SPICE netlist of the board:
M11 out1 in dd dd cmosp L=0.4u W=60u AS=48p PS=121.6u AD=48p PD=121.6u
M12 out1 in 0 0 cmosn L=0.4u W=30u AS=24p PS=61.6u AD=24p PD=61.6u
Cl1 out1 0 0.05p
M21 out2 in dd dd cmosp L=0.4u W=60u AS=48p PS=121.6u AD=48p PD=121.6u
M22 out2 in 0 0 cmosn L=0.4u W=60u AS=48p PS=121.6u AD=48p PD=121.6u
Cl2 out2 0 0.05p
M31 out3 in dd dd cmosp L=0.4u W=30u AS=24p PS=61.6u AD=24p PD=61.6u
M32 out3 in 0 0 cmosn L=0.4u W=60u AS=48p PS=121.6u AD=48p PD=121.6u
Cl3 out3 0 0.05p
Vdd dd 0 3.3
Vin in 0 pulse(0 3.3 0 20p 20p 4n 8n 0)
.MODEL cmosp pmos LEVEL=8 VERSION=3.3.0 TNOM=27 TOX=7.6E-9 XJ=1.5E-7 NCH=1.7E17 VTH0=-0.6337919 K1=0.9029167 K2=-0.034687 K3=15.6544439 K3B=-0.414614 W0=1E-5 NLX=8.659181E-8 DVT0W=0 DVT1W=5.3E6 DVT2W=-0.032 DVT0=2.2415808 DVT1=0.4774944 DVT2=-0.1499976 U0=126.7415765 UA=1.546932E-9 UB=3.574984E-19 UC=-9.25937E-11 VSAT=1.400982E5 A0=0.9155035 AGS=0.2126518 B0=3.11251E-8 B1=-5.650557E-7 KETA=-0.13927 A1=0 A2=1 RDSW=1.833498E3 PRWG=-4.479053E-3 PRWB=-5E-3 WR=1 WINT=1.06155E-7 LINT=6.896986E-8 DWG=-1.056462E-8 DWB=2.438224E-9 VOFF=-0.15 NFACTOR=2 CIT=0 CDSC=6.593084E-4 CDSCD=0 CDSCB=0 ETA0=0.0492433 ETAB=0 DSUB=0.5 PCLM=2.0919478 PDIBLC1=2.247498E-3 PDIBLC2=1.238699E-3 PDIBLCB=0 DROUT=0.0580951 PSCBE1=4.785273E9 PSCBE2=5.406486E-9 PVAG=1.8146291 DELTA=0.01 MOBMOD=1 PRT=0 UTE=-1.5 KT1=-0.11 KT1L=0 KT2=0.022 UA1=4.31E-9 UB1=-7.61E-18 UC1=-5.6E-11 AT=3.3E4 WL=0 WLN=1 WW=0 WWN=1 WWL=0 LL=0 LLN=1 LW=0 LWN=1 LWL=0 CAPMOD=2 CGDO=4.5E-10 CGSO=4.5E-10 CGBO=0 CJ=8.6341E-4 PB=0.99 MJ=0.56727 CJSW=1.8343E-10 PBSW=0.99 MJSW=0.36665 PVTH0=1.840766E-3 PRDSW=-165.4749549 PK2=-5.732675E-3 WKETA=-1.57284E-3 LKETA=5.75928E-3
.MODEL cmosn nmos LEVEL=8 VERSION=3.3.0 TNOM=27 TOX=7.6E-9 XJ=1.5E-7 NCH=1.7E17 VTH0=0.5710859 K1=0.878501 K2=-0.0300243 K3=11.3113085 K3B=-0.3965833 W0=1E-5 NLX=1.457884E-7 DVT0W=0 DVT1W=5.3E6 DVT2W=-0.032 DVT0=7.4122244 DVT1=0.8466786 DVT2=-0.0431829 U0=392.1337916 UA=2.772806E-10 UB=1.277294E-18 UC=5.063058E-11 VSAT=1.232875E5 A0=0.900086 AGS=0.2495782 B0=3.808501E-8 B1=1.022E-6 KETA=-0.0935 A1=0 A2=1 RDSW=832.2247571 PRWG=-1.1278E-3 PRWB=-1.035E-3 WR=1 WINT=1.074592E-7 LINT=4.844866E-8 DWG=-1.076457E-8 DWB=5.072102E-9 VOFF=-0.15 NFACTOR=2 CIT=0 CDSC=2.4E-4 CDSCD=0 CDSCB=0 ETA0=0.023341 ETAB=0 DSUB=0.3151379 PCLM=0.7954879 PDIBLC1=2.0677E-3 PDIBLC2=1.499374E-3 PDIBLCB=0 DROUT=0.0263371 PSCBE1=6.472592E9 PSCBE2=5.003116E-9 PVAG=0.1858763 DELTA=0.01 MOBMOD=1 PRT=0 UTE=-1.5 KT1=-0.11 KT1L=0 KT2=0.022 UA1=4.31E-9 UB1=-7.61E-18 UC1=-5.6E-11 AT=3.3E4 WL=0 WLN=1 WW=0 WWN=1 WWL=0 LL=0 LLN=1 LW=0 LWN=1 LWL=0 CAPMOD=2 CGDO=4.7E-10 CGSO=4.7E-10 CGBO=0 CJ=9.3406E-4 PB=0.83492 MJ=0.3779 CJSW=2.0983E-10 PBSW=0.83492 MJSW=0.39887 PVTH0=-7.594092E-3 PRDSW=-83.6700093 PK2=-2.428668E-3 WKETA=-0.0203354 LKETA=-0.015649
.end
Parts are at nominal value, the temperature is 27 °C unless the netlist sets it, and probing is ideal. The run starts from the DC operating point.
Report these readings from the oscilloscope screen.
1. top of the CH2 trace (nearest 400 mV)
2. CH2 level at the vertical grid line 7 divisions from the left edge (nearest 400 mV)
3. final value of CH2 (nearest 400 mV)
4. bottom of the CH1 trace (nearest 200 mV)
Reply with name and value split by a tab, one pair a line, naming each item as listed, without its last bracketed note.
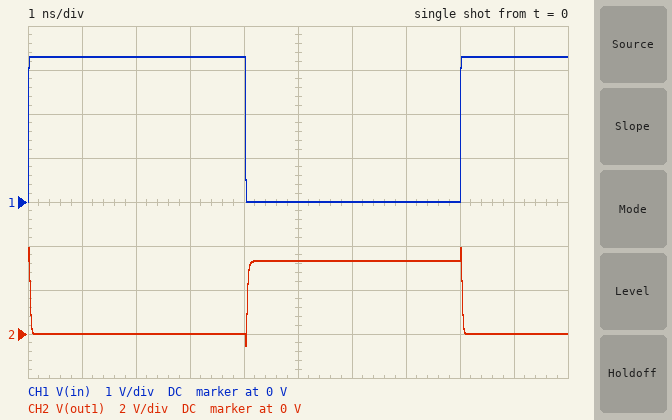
top of the CH2 trace	4.0 V
CH2 level at the vertical grid line 7 divisions from the left edge	3.2 V
final value of CH2	0 V
bottom of the CH1 trace	0 V
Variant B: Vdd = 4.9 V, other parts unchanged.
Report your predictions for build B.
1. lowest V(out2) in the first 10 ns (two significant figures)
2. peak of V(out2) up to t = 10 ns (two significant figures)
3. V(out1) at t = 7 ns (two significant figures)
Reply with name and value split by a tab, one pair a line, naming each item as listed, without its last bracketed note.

lowest V(out2) in the first 10 ns	-200 mV
peak of V(out2) up to t = 10 ns	5.4 V
V(out1) at t = 7 ns	4.9 V
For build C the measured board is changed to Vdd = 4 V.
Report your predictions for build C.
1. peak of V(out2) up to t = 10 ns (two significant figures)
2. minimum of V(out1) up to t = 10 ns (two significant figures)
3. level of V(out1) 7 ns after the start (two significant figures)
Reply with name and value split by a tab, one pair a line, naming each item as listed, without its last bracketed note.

peak of V(out2) up to t = 10 ns	4.6 V
minimum of V(out1) up to t = 10 ns	-400 mV
level of V(out1) 7 ns after the start	4.0 V
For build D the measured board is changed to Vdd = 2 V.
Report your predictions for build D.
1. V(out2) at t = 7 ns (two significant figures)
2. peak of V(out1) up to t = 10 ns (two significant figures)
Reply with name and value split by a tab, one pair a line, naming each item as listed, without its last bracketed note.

V(out2) at t = 7 ns	2.0 V
peak of V(out1) up to t = 10 ns	2.7 V
